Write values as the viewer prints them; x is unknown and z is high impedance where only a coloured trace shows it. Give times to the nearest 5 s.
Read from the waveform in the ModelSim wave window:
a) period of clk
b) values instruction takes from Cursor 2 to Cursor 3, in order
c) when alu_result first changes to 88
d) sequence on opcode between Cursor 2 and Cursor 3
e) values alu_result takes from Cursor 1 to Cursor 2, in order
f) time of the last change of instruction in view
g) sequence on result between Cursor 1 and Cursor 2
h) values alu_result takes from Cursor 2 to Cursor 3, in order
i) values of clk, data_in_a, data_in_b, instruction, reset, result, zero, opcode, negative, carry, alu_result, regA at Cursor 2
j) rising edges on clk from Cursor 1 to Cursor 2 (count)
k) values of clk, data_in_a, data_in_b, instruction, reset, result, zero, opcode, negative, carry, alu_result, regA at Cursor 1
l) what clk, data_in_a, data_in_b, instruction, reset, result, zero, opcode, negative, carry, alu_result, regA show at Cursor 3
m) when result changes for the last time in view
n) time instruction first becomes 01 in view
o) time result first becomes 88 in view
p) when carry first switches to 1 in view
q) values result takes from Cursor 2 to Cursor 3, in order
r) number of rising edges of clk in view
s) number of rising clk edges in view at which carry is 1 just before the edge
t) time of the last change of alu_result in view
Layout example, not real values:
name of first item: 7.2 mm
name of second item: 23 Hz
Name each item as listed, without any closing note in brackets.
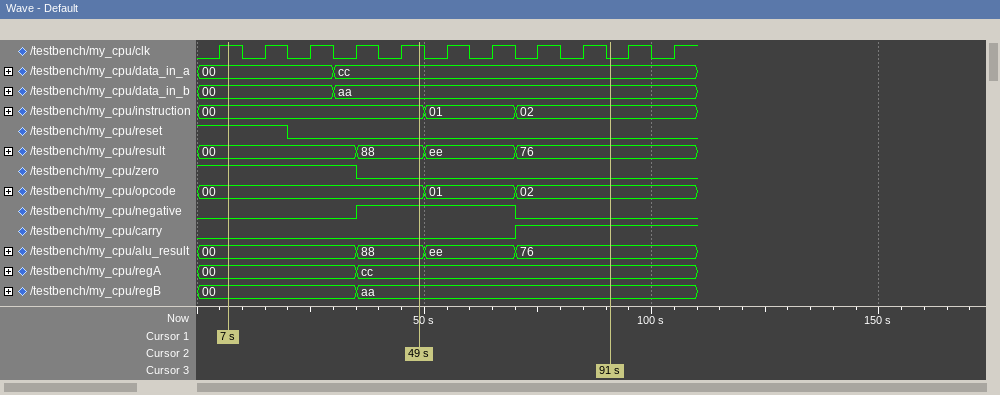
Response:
period of clk: 10 s
values instruction takes from Cursor 2 to Cursor 3, in order: 00, 01, 02
when alu_result first changes to 88: 35 s
sequence on opcode between Cursor 2 and Cursor 3: 00, 01, 02
values alu_result takes from Cursor 1 to Cursor 2, in order: 00, 88
time of the last change of instruction in view: 70 s
sequence on result between Cursor 1 and Cursor 2: 00, 88
values alu_result takes from Cursor 2 to Cursor 3, in order: 88, ee, 76
values of clk, data_in_a, data_in_b, instruction, reset, result, zero, opcode, negative, carry, alu_result, regA at Cursor 2: clk=1, data_in_a=cc, data_in_b=aa, instruction=00, reset=0, result=88, zero=0, opcode=00, negative=1, carry=0, alu_result=88, regA=cc
rising edges on clk from Cursor 1 to Cursor 2: 4
values of clk, data_in_a, data_in_b, instruction, reset, result, zero, opcode, negative, carry, alu_result, regA at Cursor 1: clk=1, data_in_a=00, data_in_b=00, instruction=00, reset=1, result=00, zero=1, opcode=00, negative=0, carry=0, alu_result=00, regA=00
what clk, data_in_a, data_in_b, instruction, reset, result, zero, opcode, negative, carry, alu_result, regA show at Cursor 3: clk=0, data_in_a=cc, data_in_b=aa, instruction=02, reset=0, result=76, zero=0, opcode=02, negative=0, carry=1, alu_result=76, regA=cc
when result changes for the last time in view: 70 s
time instruction first becomes 01 in view: 50 s
time result first becomes 88 in view: 35 s
when carry first switches to 1 in view: 70 s
values result takes from Cursor 2 to Cursor 3, in order: 88, ee, 76
number of rising edges of clk in view: 11
number of rising clk edges in view at which carry is 1 just before the edge: 4
time of the last change of alu_result in view: 70 s
